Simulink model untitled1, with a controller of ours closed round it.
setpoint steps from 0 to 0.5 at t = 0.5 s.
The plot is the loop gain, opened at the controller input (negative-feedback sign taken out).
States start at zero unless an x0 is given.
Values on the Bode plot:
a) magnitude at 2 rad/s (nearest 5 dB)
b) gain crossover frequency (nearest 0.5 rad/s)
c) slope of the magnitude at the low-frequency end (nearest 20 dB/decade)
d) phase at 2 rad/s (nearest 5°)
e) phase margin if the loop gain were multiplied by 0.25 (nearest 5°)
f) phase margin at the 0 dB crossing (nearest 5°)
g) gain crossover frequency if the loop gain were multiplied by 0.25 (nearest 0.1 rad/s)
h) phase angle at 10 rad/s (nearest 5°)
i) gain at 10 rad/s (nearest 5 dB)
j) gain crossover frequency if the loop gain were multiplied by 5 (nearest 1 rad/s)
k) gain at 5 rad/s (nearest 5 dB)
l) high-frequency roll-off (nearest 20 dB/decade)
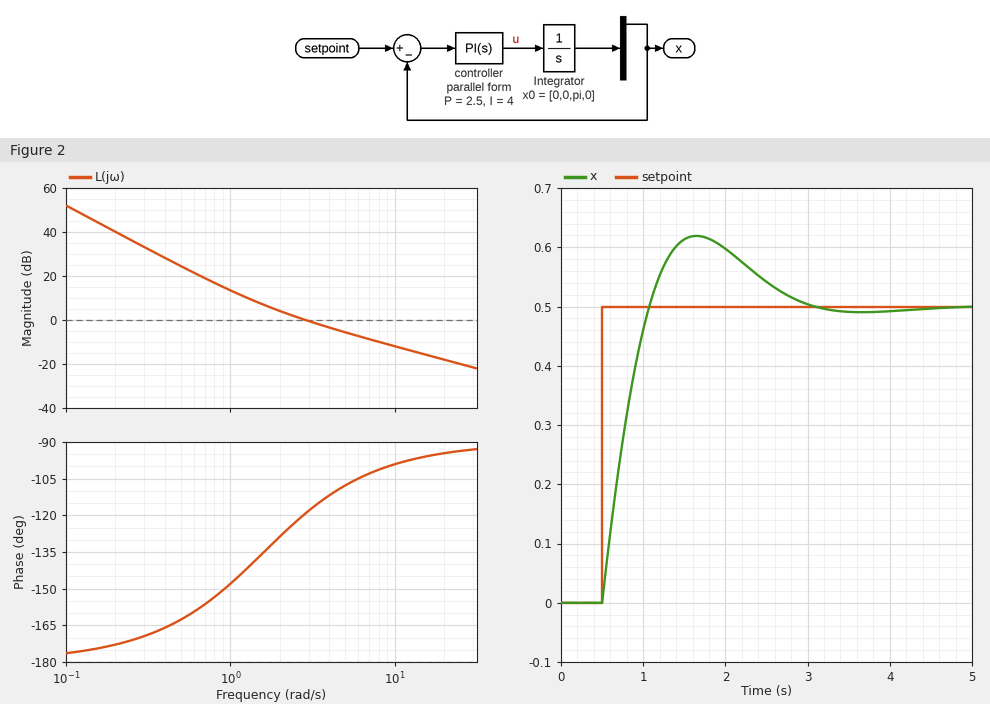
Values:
5 dB
3.0 rad/s
-40 dB/decade
-130°
35°
60°
1.1 rad/s
-100°
-10 dB
13 rad/s
-5 dB
-20 dB/decade
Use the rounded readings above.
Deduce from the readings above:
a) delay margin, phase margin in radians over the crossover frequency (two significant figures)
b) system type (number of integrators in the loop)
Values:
0.35 s
2
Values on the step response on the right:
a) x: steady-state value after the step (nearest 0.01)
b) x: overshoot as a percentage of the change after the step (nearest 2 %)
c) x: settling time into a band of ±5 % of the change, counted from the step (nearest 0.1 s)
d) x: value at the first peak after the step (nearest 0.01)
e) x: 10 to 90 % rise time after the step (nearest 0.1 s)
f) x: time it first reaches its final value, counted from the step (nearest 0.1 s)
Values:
0.50
24 %
2.2 s
0.62
0.4 s
0.6 s
